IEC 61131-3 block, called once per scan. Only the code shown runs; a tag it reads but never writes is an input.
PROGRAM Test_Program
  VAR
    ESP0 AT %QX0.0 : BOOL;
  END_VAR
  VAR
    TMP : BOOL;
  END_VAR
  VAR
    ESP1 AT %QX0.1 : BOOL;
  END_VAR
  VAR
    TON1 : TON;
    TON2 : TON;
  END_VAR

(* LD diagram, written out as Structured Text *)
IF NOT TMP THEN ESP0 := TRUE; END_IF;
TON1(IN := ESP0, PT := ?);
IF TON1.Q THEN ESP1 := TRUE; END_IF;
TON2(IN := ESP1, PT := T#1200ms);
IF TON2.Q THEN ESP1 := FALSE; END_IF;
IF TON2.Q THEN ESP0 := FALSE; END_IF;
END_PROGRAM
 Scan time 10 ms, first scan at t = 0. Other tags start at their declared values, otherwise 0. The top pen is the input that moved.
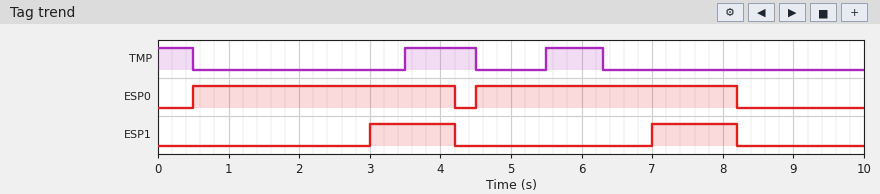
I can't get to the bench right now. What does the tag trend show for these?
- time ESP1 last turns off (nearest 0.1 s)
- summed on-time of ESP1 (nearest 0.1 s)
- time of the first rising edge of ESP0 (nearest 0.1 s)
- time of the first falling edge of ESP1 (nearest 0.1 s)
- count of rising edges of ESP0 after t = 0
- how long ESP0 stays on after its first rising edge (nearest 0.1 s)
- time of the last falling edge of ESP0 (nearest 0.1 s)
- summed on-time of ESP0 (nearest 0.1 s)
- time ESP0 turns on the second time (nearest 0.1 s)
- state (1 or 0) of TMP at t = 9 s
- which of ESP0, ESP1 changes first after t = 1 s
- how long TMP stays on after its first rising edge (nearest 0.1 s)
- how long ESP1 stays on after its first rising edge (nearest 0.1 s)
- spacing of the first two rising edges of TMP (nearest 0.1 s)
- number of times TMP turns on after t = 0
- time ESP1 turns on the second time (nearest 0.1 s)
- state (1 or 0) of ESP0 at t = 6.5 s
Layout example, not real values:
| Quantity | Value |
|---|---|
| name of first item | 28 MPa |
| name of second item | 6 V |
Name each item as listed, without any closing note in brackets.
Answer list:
| Quantity | Value |
|---|---|
| time ESP1 last turns off | 8.2 s |
| summed on-time of ESP1 | 2.4 s |
| time of the first rising edge of ESP0 | 0.5 s |
| time of the first falling edge of ESP1 | 4.2 s |
| count of rising edges of ESP0 after t = 0 | 2 |
| how long ESP0 stays on after its first rising edge | 3.7 s |
| time of the last falling edge of ESP0 | 8.2 s |
| summed on-time of ESP0 | 7.4 s |
| time ESP0 turns on the second time | 4.5 s |
| state (1 or 0) of TMP at t = 9 s | 0 |
| which of ESP0, ESP1 changes first after t = 1 s | ESP1 |
| how long TMP stays on after its first rising edge | 1.0 s |
| how long ESP1 stays on after its first rising edge | 1.2 s |
| spacing of the first two rising edges of TMP | 2.0 s |
| number of times TMP turns on after t = 0 | 2 |
| time ESP1 turns on the second time | 7.0 s |
| state (1 or 0) of ESP0 at t = 6.5 s | 1 |
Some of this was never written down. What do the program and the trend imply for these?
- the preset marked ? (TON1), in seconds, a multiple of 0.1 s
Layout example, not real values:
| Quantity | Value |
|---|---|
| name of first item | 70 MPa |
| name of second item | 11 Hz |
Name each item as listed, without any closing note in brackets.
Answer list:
| Quantity | Value |
|---|---|
| the preset marked ? (TON1), in seconds, a multiple of 0.1 s | 2.5 s |
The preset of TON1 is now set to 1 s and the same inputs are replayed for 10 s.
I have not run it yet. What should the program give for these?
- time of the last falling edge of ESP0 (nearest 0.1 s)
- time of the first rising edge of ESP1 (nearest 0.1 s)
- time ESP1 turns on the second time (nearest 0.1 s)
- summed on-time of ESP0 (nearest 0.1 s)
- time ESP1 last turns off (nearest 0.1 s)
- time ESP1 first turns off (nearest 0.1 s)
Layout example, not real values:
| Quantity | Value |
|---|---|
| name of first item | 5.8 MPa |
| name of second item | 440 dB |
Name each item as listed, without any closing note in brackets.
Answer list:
| Quantity | Value |
|---|---|
| time of the last falling edge of ESP0 | 6.7 s |
| time of the first rising edge of ESP1 | 1.5 s |
| time ESP1 turns on the second time | 5.5 s |
| summed on-time of ESP0 | 4.4 s |
| time ESP1 last turns off | 6.7 s |
| time ESP1 first turns off | 2.7 s |
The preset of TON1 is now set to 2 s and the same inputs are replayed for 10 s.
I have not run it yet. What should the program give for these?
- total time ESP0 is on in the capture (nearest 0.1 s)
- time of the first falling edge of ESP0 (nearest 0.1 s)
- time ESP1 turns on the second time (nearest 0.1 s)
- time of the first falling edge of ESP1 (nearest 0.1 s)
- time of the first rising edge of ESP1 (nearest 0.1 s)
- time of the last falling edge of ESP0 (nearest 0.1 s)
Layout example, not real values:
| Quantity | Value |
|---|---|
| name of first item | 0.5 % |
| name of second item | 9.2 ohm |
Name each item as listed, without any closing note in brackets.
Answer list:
| Quantity | Value |
|---|---|
| total time ESP0 is on in the capture | 6.4 s |
| time of the first falling edge of ESP0 | 3.7 s |
| time ESP1 turns on the second time | 6.5 s |
| time of the first falling edge of ESP1 | 3.7 s |
| time of the first rising edge of ESP1 | 2.5 s |
| time of the last falling edge of ESP0 | 7.7 s |
